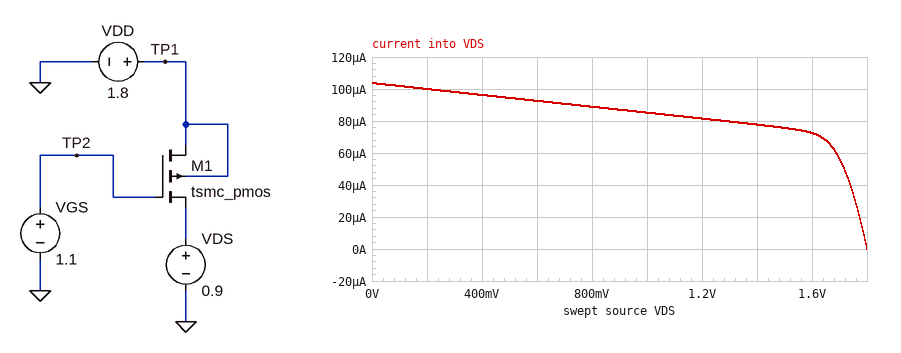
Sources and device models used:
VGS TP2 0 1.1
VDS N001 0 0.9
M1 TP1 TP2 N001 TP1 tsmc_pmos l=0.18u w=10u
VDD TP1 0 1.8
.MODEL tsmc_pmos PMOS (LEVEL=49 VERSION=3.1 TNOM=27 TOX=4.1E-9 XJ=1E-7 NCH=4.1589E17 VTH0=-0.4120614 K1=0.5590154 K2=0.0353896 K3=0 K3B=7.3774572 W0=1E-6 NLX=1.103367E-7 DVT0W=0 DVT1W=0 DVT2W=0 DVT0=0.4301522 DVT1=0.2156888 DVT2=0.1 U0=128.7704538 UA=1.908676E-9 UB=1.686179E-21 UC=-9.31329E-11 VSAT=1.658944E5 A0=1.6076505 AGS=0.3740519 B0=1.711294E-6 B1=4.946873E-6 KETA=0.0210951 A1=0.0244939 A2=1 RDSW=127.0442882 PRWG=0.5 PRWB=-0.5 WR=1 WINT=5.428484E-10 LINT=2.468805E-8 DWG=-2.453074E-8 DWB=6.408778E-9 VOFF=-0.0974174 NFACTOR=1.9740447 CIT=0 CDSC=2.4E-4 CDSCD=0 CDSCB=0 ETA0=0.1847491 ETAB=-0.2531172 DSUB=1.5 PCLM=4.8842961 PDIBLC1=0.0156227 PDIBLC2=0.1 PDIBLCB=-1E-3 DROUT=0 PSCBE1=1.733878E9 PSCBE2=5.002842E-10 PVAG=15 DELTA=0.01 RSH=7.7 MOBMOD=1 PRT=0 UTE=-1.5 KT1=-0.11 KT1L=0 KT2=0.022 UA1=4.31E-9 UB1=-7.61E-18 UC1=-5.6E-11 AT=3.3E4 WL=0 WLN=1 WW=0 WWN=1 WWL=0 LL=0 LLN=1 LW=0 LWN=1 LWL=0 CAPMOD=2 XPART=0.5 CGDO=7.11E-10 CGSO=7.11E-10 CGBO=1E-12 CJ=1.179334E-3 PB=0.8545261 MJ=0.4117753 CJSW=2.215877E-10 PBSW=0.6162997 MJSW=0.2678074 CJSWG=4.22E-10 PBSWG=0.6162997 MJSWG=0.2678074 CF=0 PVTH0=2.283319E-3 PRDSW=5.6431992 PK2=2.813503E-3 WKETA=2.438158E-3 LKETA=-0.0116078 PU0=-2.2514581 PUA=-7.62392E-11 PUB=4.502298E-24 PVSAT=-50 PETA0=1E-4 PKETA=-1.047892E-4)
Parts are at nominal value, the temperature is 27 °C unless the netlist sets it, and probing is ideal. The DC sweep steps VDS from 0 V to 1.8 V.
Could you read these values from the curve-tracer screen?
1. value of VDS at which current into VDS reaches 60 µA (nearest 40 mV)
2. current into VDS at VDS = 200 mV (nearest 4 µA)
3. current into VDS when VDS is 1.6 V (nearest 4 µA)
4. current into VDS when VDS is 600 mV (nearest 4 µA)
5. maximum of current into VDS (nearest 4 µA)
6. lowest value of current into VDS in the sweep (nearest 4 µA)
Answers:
1.68 V
100 µA
72 µA
92 µA
104 µA
0 A
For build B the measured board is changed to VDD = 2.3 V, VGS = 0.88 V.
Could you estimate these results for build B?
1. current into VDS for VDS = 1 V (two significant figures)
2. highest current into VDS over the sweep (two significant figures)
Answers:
1.4 mA
1.5 mA
